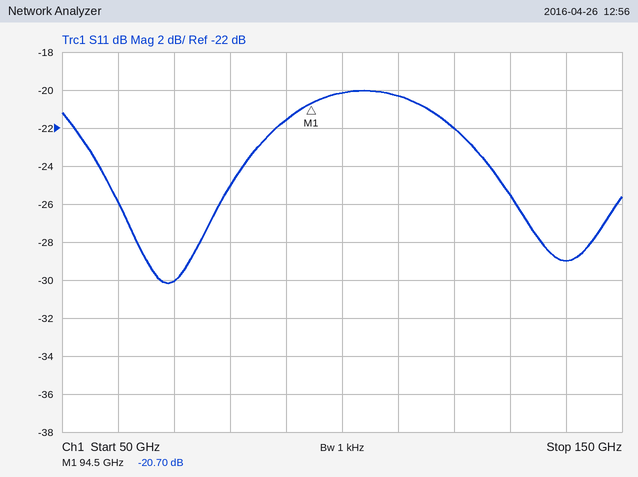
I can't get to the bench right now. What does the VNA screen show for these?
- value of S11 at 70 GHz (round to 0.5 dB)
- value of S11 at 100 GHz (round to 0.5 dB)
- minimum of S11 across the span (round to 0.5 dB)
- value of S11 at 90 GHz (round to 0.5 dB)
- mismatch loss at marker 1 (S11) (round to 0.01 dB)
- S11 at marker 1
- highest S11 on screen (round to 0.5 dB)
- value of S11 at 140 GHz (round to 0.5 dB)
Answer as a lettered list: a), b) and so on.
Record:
a) -30.0 dB
b) -20.0 dB
c) -30.0 dB
d) -21.5 dB
e) 0.04 dB
f) -20.70 dB
g) -20.0 dB
h) -29.0 dB
